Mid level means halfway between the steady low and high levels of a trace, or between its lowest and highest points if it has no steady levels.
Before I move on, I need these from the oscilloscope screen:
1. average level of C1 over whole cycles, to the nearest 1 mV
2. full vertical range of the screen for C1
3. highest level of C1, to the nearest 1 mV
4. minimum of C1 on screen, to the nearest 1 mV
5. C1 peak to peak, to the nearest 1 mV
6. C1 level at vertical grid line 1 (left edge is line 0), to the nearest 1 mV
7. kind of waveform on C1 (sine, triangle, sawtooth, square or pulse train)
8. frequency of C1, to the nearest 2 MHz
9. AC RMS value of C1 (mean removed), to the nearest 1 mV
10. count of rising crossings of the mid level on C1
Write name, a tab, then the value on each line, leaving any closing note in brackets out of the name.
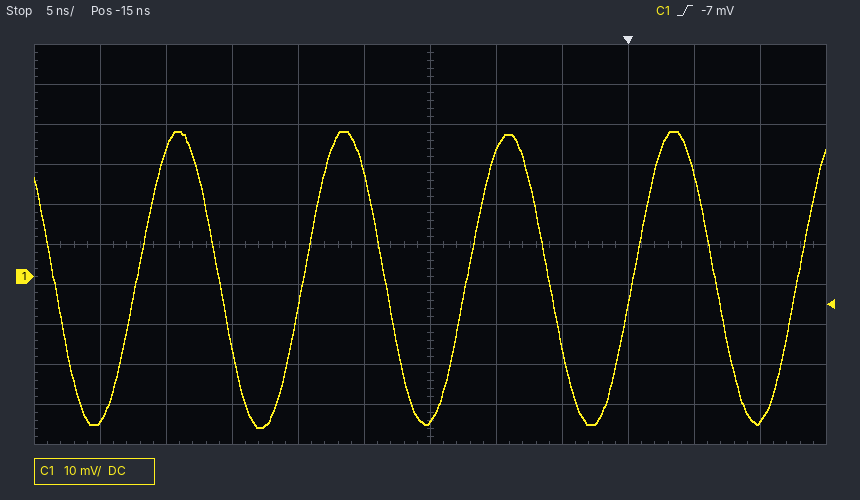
average level of C1 over whole cycles, to the nearest 1 mV	-1 mV
full vertical range of the screen for C1	100 mV
highest level of C1, to the nearest 1 mV	36 mV
minimum of C1 on screen, to the nearest 1 mV	-38 mV
C1 peak to peak, to the nearest 1 mV	74 mV
C1 level at vertical grid line 1 (left edge is line 0), to the nearest 1 mV	-36 mV
kind of waveform on C1	sine
frequency of C1, to the nearest 2 MHz	80 MHz
AC RMS value of C1 (mean removed), to the nearest 1 mV	26 mV
count of rising crossings of the mid level on C1	5
